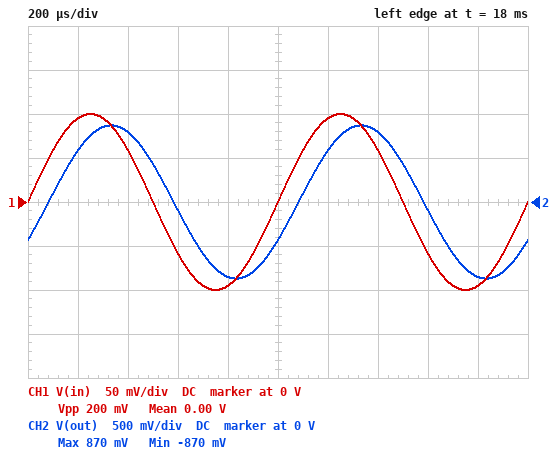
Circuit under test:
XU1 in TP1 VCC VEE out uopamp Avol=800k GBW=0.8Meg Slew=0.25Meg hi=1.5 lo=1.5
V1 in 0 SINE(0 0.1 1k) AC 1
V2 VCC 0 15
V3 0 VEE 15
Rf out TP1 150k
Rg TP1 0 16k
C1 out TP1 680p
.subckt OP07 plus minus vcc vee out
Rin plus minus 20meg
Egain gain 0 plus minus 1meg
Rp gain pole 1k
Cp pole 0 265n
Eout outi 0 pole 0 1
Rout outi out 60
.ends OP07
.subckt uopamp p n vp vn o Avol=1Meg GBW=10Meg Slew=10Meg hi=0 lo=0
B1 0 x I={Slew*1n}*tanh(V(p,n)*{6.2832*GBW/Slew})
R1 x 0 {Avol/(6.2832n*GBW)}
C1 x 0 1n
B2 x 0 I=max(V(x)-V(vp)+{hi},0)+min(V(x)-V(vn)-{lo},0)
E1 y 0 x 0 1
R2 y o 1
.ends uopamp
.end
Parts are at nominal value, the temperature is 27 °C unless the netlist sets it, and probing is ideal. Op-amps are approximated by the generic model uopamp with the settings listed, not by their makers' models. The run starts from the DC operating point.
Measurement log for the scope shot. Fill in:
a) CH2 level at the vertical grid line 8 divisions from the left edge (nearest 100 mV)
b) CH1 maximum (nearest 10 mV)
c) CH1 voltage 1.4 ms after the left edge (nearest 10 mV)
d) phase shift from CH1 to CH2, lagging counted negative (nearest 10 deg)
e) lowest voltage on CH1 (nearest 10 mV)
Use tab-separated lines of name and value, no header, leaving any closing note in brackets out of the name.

CH2 level at the vertical grid line 8 divisions from the left edge	-100 mV
CH1 maximum	100 mV
CH1 voltage 1.4 ms after the left edge	60 mV
phase shift from CH1 to CH2, lagging counted negative	-30 deg
lowest voltage on CH1	-100 mV
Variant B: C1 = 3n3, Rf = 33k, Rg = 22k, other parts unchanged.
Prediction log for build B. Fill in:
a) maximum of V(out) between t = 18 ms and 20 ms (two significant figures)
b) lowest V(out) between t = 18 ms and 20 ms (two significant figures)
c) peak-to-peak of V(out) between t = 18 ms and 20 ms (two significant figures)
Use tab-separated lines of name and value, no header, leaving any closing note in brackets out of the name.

maximum of V(out) between t = 18 ms and 20 ms	210 mV
lowest V(out) between t = 18 ms and 20 ms	-210 mV
peak-to-peak of V(out) between t = 18 ms and 20 ms	430 mV
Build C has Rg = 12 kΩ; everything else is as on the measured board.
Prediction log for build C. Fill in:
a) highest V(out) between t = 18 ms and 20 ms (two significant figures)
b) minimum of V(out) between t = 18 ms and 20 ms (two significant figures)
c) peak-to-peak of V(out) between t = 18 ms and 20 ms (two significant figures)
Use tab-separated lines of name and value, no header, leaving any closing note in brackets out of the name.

highest V(out) between t = 18 ms and 20 ms	1.1 V
minimum of V(out) between t = 18 ms and 20 ms	-1.1 V
peak-to-peak of V(out) between t = 18 ms and 20 ms	2.3 V
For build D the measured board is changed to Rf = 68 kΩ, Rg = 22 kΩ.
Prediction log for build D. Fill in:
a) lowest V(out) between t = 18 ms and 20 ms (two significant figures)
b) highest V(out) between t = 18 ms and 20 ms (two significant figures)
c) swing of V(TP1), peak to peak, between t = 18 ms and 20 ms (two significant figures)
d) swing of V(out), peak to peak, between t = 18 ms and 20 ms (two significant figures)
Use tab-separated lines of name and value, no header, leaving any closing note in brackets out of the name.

lowest V(out) between t = 18 ms and 20 ms	-390 mV
highest V(out) between t = 18 ms and 20 ms	390 mV
swing of V(TP1), peak to peak, between t = 18 ms and 20 ms	200 mV
swing of V(out), peak to peak, between t = 18 ms and 20 ms	790 mV
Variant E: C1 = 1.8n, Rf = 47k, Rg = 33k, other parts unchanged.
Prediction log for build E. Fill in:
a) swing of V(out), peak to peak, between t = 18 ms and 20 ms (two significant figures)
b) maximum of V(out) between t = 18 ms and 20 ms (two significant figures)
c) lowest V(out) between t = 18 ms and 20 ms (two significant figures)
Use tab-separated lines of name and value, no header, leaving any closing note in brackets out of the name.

swing of V(out), peak to peak, between t = 18 ms and 20 ms	440 mV
maximum of V(out) between t = 18 ms and 20 ms	220 mV
lowest V(out) between t = 18 ms and 20 ms	-220 mV
